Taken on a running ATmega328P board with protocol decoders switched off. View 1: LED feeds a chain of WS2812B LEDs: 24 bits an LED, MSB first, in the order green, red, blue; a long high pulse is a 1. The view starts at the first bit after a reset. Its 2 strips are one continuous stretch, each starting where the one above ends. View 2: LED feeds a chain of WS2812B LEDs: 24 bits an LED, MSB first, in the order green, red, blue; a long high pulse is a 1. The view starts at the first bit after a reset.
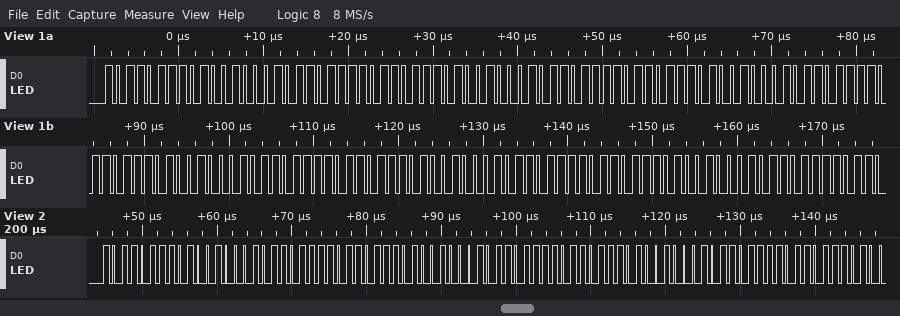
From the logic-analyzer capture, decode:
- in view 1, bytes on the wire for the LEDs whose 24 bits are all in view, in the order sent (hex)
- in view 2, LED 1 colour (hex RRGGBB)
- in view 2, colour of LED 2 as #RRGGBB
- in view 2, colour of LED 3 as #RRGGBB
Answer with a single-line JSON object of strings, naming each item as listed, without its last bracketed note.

{"in view 1, bytes on the wire for the LEDs whose 24 bits are all in view, in the order sent": "B7 48 B7 B7 48 B7 B7 48 B7 B7 48 B7 B7 48 B7 B7 48 B7", "in view 2, LED 1 colour": "#48B7B7", "in view 2, colour of LED 2 as #RRGGBB": "#48B7B7", "in view 2, colour of LED 3 as #RRGGBB": "#48B7B7"}
